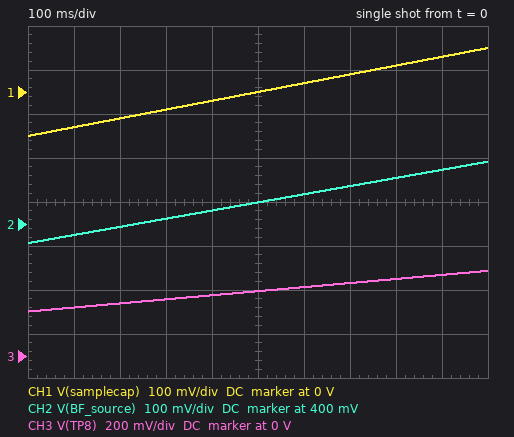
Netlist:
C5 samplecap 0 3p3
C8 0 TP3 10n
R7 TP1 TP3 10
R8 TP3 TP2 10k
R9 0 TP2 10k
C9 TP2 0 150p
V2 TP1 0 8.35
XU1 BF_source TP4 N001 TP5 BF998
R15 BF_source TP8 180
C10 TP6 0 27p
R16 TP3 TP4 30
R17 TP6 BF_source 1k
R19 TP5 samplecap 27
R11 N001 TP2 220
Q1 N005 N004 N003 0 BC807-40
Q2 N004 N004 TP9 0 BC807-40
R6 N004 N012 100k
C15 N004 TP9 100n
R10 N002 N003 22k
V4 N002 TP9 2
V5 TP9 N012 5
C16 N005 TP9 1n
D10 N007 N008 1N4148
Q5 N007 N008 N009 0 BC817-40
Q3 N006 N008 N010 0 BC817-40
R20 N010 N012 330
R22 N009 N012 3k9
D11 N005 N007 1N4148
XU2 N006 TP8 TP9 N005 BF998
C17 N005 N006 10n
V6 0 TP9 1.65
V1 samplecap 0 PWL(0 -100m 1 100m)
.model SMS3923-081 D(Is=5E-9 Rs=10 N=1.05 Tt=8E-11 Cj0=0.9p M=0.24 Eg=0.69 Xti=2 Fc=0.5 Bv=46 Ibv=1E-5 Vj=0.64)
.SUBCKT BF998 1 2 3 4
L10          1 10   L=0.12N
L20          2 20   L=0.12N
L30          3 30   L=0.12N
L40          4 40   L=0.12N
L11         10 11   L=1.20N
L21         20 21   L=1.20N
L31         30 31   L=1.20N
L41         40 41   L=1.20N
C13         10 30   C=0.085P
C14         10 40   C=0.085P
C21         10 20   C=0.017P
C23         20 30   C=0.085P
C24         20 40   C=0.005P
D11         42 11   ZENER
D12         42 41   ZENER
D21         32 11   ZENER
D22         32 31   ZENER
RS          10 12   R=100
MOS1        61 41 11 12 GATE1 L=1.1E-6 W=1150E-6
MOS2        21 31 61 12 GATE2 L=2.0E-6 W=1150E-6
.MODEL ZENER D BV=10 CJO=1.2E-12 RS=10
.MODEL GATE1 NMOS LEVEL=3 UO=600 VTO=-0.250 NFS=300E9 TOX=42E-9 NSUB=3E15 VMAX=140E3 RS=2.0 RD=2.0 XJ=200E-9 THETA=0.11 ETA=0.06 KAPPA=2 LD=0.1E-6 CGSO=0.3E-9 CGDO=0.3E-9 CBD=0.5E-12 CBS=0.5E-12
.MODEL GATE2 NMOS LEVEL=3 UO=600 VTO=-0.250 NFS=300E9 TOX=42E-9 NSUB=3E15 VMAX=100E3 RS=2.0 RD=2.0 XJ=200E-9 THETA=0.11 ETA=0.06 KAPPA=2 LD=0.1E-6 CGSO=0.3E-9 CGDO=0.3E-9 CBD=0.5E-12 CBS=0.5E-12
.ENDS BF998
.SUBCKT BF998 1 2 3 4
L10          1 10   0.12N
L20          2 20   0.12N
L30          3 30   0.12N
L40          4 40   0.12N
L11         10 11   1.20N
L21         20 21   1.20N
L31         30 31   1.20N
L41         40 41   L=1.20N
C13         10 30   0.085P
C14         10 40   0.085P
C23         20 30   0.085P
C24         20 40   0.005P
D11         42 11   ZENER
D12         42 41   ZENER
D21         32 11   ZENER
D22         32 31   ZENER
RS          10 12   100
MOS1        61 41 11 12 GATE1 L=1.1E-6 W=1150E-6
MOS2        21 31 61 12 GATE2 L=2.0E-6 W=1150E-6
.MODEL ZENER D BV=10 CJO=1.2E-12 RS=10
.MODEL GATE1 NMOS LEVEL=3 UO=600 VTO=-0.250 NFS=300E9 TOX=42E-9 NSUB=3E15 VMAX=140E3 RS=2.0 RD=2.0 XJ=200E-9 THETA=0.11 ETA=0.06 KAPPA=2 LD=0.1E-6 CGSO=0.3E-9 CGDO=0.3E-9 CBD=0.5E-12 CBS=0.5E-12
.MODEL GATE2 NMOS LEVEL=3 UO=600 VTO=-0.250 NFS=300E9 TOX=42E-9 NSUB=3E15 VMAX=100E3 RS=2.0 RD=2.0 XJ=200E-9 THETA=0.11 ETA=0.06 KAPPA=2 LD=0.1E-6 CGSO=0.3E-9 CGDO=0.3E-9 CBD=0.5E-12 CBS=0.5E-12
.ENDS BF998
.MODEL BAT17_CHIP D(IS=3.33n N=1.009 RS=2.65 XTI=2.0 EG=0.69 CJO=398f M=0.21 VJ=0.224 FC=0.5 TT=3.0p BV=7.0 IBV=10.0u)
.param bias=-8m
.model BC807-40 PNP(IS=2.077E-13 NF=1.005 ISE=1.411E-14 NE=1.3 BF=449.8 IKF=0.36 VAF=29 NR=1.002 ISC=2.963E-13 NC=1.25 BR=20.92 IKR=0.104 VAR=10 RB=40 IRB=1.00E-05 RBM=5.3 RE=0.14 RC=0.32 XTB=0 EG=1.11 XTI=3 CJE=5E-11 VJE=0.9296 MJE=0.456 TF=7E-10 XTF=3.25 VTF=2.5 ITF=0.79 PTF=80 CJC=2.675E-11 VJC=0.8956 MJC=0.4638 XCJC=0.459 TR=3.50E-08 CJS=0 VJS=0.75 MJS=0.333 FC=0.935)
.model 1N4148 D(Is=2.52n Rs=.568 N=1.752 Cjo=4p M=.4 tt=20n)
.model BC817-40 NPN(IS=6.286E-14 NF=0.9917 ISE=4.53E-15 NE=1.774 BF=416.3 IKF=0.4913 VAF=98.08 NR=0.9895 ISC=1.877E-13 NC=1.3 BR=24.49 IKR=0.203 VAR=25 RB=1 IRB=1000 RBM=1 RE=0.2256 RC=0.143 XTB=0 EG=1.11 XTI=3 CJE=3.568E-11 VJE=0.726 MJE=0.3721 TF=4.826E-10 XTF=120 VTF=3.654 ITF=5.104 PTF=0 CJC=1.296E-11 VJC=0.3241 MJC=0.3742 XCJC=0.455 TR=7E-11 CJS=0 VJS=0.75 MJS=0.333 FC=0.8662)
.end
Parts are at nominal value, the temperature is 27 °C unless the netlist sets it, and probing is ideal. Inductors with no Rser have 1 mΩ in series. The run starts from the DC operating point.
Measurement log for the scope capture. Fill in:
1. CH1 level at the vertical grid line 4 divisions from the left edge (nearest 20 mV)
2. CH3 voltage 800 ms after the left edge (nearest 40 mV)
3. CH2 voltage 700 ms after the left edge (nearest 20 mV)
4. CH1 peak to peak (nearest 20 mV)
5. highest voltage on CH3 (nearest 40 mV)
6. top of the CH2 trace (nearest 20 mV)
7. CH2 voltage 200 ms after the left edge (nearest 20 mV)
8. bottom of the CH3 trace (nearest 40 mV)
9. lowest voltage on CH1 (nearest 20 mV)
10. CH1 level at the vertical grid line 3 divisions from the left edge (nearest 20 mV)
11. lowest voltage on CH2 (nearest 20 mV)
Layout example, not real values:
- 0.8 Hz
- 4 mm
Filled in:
- -20 mV
- 360 mV
- 480 mV
- 200 mV
- 400 mV
- 540 mV
- 400 mV
- 200 mV
- -100 mV
- -40 mV
- 360 mV
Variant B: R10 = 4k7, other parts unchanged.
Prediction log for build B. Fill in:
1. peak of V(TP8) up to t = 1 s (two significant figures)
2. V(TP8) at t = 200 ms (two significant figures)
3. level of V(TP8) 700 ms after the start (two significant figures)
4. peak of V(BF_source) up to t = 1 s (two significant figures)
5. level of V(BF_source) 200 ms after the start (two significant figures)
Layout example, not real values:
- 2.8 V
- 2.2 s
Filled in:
- -520 mV
- -660 mV
- -570 mV
- 300 mV
- 150 mV
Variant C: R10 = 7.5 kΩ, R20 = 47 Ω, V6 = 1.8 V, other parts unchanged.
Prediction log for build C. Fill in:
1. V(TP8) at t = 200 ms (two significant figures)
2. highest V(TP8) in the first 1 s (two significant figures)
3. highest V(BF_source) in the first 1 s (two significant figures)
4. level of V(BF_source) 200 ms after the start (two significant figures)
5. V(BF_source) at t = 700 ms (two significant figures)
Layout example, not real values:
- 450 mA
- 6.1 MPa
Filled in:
- -3.1 V
- -3.0 V
- -120 mV
- -260 mV
- -170 mV
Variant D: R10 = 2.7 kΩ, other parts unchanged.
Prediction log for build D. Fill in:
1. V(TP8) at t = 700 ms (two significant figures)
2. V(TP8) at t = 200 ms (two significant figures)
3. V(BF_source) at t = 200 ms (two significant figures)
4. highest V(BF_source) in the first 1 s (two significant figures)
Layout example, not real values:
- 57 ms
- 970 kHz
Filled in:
- -1.3 V
- -1.4 V
- 6.7 mV
- 150 mV
